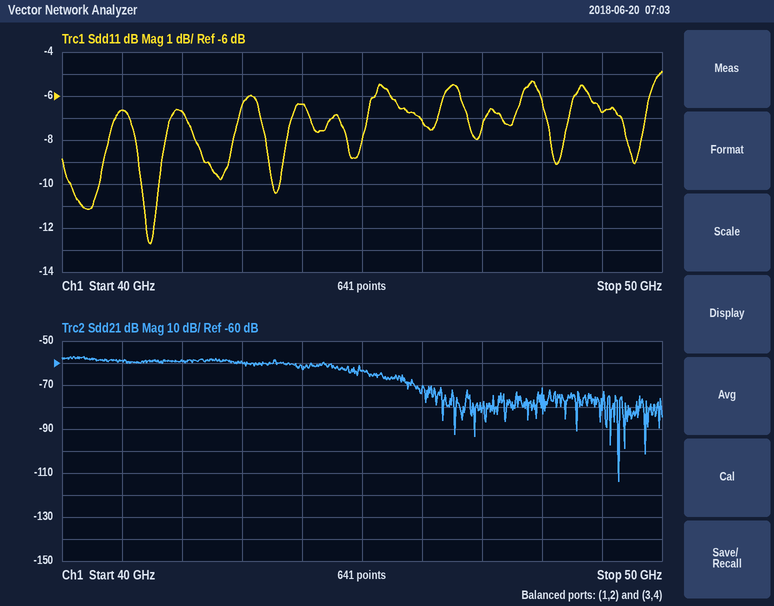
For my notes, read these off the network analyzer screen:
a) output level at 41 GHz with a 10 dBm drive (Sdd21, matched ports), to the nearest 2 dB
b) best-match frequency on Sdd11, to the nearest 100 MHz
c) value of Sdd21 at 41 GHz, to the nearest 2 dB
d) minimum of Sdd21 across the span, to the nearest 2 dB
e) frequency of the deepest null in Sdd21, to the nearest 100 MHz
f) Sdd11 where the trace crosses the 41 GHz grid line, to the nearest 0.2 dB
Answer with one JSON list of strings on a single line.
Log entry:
["-48 dBm", "41.5 GHz", "-58 dB", "-114 dB", "49.3 GHz", "-6.6 dB"]
